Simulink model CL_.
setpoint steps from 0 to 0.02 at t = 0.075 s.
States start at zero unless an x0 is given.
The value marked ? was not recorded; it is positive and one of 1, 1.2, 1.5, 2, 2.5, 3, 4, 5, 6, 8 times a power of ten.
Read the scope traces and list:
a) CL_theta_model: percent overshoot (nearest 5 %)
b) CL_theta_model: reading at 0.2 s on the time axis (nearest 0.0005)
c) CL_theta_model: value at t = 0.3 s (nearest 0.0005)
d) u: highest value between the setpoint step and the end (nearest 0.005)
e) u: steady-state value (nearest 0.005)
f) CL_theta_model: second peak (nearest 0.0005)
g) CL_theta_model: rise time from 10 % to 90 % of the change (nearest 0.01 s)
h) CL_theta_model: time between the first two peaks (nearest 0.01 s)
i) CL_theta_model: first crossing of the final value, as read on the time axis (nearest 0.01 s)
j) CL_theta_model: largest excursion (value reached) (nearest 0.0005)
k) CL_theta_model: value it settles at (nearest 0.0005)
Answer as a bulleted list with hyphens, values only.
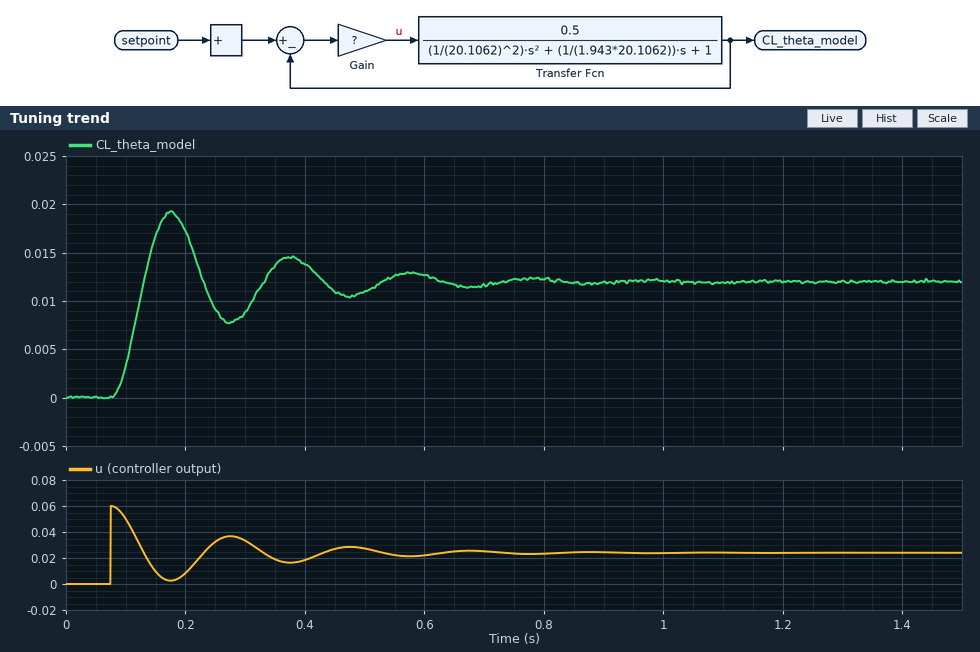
- 60 %
- 0.0170
- 0.0090
- 0.060
- 0.025
- 0.0145
- 0.04 s
- 0.20 s
- 0.13 s
- 0.0190
- 0.0120
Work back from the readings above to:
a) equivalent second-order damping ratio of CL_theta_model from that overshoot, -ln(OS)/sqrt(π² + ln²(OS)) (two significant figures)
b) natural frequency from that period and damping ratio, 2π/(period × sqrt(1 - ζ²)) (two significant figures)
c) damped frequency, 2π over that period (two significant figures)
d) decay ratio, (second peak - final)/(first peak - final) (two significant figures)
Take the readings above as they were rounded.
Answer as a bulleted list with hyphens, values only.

- 0.16
- 32 rad/s
- 31 rad/s
- 0.36
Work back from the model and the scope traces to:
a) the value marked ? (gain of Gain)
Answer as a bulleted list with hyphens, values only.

- 3
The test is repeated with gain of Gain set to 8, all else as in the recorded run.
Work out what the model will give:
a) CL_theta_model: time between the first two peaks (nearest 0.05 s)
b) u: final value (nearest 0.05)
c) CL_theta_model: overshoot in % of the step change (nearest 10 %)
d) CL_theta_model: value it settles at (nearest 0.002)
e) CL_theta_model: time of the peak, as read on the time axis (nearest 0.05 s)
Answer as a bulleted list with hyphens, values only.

- 0.15 s
- 0.05
- 70 %
- 0.016
- 0.15 s
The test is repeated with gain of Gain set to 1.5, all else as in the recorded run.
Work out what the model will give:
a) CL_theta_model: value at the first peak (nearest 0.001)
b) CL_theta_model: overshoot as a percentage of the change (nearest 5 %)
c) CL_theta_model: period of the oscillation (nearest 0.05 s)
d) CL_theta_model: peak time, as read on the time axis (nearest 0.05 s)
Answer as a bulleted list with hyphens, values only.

- 0.013
- 55 %
- 0.25 s
- 0.20 s
